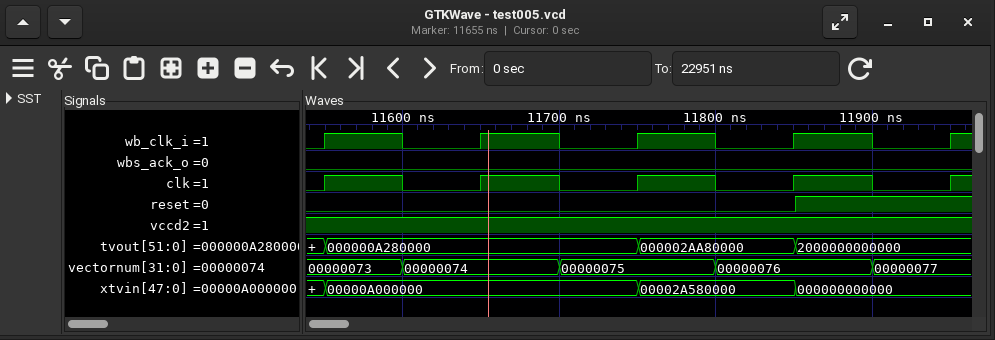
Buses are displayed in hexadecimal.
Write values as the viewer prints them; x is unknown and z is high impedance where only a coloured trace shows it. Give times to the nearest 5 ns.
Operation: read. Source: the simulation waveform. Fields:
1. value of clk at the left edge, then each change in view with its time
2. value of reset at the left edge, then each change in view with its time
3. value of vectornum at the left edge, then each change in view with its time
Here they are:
0, 1 at 11550 ns, 0 at 11600 ns, 1 at 11650 ns, 0 at 11700 ns, 1 at 11750 ns, 0 at 11800 ns, 1 at 11850 ns, 0 at 11900 ns, 1 at 11950 ns
0, 1 at 11850 ns
00000073, 00000074 at 11600 ns, 00000075 at 11700 ns, 00000076 at 11800 ns, 00000077 at 11900 ns
